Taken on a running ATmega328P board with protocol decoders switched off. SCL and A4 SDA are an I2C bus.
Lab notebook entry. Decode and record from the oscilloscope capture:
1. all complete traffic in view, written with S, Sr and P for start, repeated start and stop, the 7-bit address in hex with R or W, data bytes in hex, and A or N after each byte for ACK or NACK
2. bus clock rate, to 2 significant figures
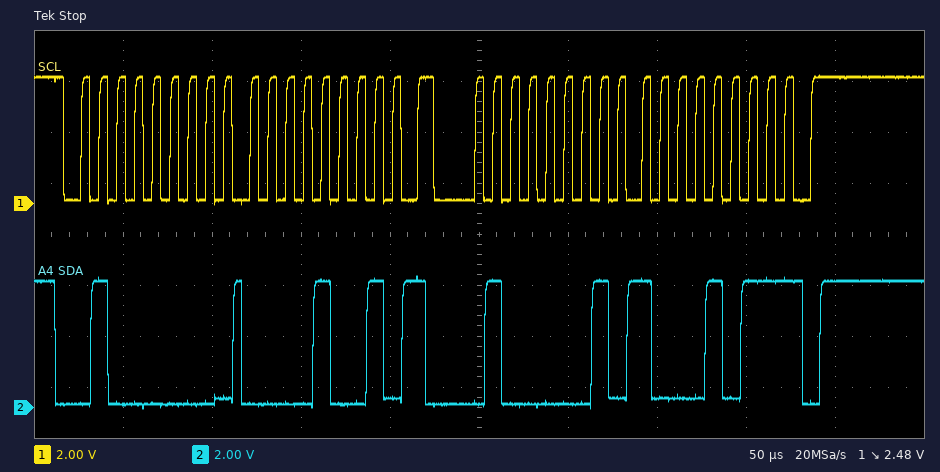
S 20W A 09 A Sr 20R A 8B N P
100 kHz
